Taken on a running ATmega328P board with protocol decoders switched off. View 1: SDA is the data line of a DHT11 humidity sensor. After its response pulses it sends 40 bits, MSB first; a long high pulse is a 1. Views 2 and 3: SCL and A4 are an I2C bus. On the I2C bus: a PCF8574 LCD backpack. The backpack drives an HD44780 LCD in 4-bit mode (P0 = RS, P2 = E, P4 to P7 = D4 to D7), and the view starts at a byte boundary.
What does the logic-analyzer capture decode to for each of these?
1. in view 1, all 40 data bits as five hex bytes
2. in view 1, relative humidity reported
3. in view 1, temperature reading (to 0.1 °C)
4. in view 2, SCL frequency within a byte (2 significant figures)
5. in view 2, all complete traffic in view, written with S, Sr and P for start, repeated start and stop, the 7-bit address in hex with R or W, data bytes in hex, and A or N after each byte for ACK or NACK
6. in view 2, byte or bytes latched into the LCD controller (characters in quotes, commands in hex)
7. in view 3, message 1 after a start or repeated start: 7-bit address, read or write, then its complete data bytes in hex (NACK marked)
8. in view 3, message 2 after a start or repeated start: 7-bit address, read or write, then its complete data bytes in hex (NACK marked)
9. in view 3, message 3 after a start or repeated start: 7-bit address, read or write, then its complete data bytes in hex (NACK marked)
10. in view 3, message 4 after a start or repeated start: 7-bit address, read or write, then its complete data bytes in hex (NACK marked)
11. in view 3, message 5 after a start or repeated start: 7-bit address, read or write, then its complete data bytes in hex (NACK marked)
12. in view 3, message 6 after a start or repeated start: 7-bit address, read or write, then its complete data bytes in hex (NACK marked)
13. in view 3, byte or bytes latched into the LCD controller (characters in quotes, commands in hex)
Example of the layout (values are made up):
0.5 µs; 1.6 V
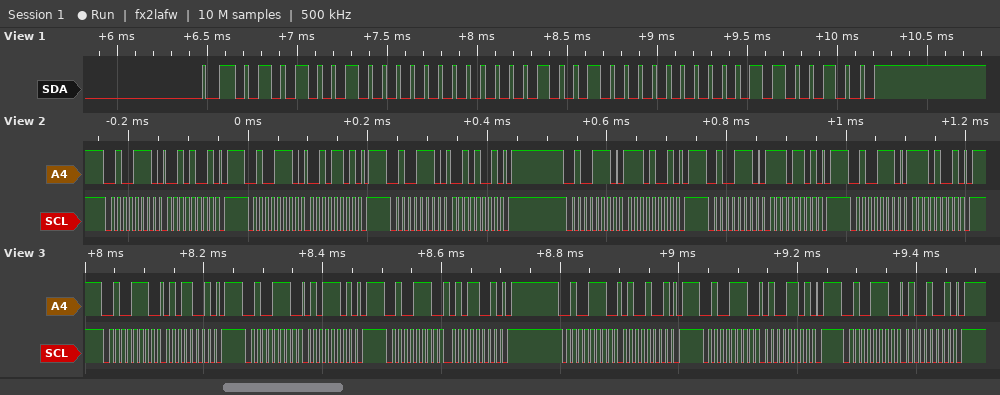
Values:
52 00 12 00 64; 82 %; 18.0 °C; 100 kHz; S 27W A 29 A P S 27W A 2D A P S 27W A 29 A P S 27W A E9 A P S 27W A ED A P S 27W A E9 A P; '.'; 0x27 write: 59; 0x27 write: 5D; 0x27 write: 59; 0x27 write: 49; 0x27 write: 4D; 0x27 write: 49; 'T'
